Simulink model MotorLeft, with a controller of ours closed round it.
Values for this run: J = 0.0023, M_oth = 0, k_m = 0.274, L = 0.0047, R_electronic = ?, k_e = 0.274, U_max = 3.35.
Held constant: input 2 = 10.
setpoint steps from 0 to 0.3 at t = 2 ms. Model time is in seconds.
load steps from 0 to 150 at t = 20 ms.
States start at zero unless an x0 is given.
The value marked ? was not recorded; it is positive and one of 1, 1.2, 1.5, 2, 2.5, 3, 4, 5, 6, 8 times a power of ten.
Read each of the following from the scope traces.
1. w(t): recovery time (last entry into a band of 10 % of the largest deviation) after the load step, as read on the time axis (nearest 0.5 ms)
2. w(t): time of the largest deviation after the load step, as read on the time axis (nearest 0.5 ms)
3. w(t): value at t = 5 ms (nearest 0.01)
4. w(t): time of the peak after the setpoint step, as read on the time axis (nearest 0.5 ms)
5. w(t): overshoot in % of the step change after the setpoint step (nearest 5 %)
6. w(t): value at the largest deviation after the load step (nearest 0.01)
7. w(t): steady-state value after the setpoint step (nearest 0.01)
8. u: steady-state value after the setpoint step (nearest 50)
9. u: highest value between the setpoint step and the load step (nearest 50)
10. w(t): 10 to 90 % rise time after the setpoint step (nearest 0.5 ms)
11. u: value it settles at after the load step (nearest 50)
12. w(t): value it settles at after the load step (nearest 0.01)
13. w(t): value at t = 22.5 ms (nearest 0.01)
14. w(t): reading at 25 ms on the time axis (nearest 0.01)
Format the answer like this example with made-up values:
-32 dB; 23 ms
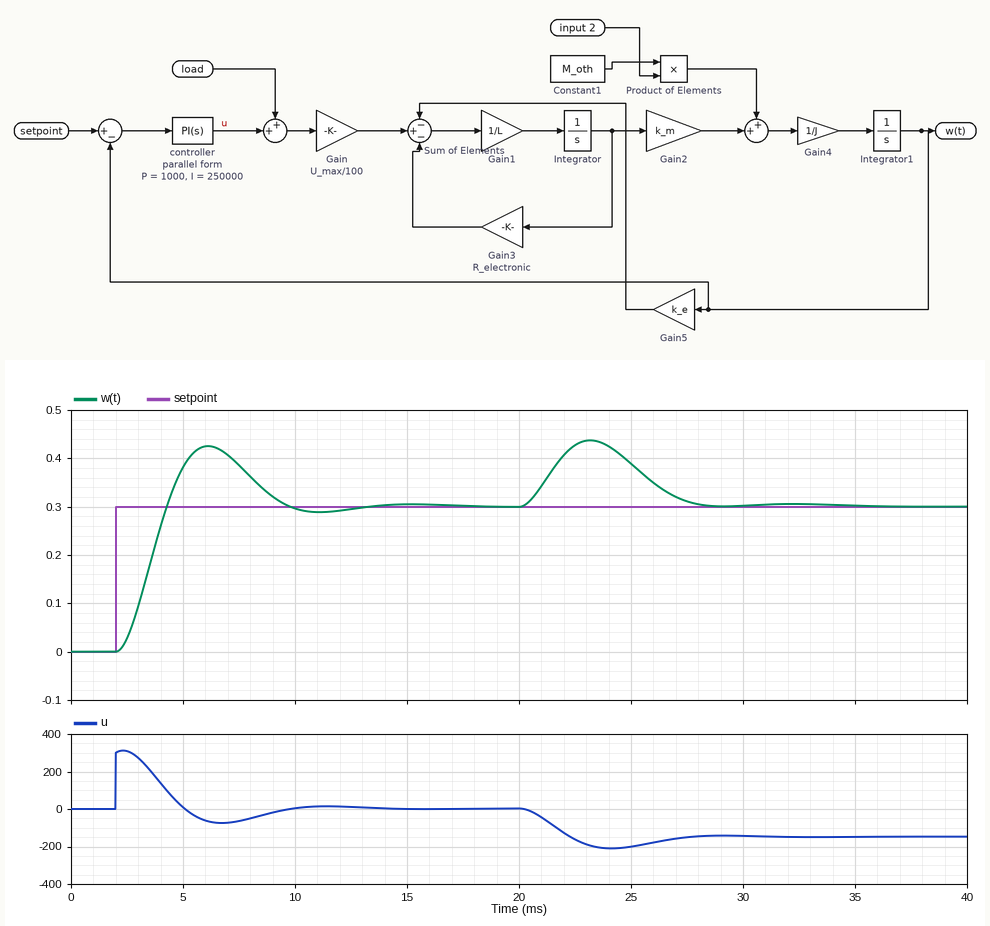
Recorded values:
27.5 ms; 23.0 ms; 0.38; 6.0 ms; 40 %; 0.44; 0.30; 0; 300; 1.5 ms; -150; 0.30; 0.43; 0.39
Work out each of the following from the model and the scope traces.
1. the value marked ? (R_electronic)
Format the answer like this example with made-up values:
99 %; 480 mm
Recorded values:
5
